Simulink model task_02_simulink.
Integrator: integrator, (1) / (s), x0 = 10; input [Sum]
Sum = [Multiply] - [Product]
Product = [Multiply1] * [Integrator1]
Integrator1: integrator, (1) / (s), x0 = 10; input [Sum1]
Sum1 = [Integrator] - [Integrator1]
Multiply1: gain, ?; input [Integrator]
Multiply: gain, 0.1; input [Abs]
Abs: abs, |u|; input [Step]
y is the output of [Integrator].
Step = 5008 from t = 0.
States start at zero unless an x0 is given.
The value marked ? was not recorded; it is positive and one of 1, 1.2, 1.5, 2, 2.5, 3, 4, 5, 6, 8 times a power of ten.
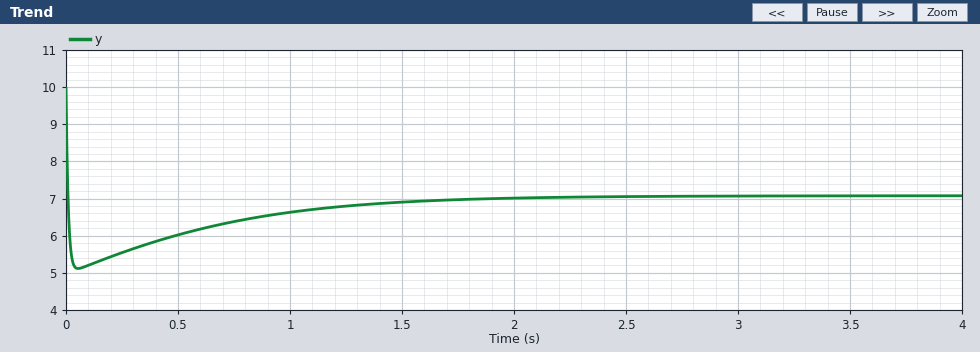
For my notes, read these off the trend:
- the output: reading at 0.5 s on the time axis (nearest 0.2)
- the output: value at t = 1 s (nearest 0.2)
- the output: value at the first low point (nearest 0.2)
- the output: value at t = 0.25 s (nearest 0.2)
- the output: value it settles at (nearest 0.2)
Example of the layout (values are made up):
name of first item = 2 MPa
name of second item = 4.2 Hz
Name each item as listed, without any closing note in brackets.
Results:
the output: reading at 0.5 s on the time axis = 6.0
the output: value at t = 1 s = 6.6
the output: value at the first low point = 5.2
the output: value at t = 0.25 s = 5.6
the output: value it settles at = 7.0
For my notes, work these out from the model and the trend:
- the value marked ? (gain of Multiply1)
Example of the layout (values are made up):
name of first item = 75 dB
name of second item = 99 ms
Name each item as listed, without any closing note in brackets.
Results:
the value marked ? = 10
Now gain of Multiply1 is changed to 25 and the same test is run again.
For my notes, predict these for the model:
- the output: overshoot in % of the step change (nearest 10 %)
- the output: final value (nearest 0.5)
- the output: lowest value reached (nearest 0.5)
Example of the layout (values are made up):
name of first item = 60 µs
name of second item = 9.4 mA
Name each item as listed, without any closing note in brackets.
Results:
the output: overshoot in % of the step change = 40 %
the output: final value = 4.5
the output: lowest value reached = 2.0
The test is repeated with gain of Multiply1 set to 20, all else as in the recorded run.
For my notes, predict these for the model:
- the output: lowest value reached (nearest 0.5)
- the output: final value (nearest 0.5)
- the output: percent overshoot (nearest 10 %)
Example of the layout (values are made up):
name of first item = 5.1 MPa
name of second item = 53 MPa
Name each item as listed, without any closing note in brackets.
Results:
the output: lowest value reached = 2.5
the output: final value = 5.0
the output: percent overshoot = 50 %
